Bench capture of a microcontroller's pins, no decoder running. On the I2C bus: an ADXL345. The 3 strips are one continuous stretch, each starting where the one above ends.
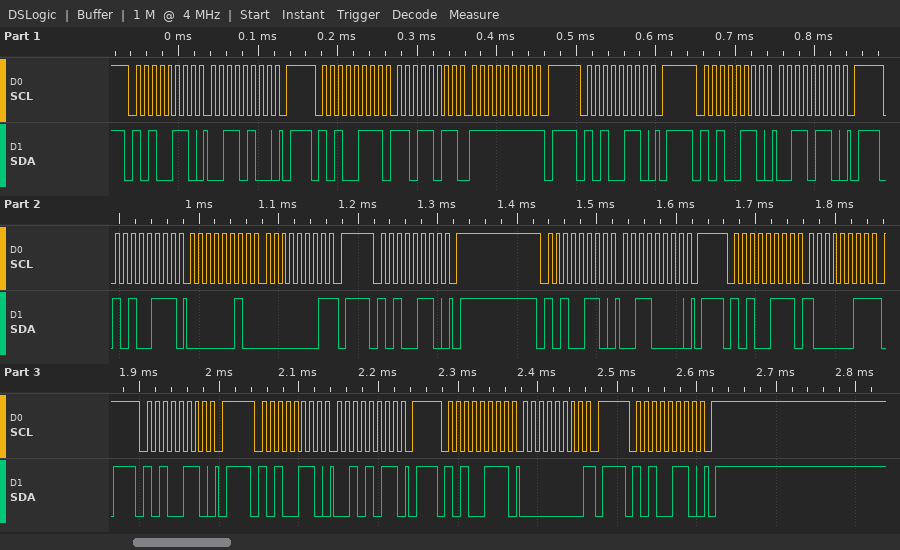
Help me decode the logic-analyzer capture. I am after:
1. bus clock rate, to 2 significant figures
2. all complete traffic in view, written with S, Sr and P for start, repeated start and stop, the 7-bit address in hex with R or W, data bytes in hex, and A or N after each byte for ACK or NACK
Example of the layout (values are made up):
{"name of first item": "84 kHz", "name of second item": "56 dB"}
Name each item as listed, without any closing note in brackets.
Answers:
{"bus clock rate, to 2 significant figures": "100 kHz", "all complete traffic in view, written with S, Sr and P for start, repeated start and stop, the 7-bit address in hex with R or W, data bytes in hex, and A or N after each byte for ACK or NACK": "S 53W A 34 A P S 53R A DB A FF N P S 53W A P S 53W A 36 A P S 53R A 02 A 01 N P S 53W A P S 53W A 30 A P S 53R A 83 N P S 53W A P S 53W A 2B A P S 53R A 00 N P S 53W A P"}
